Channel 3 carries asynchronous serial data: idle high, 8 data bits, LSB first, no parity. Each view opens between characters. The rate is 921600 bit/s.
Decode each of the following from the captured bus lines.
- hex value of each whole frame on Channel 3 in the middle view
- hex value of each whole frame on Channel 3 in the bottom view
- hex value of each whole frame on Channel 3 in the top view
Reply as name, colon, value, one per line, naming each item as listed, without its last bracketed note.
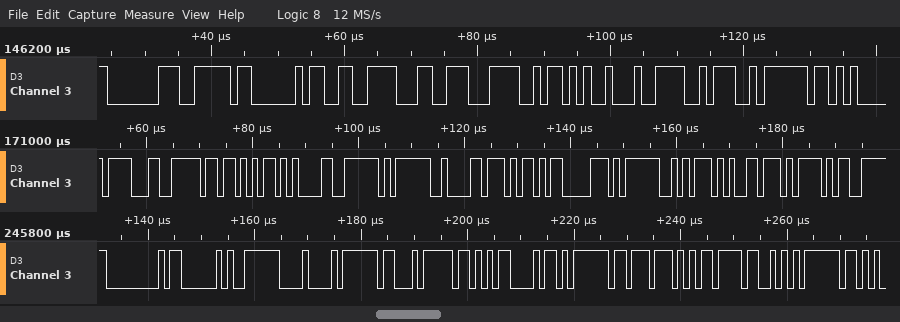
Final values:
hex value of each whole frame on Channel 3 in the middle view: 8F, BE, AB, 85, 7E, 3F, D8, AD, 70, 3F, 5D, 76, AF
hex value of each whole frame on Channel 3 in the bottom view: 00, 03, F9, 08, BF, F4, AB, 68, BF, 77, ED, 53, BF
hex value of each whole frame on Channel 3 in the top view: C0, BE, A0, E6, CC, 3C, 2B, E4, 3A, BF
